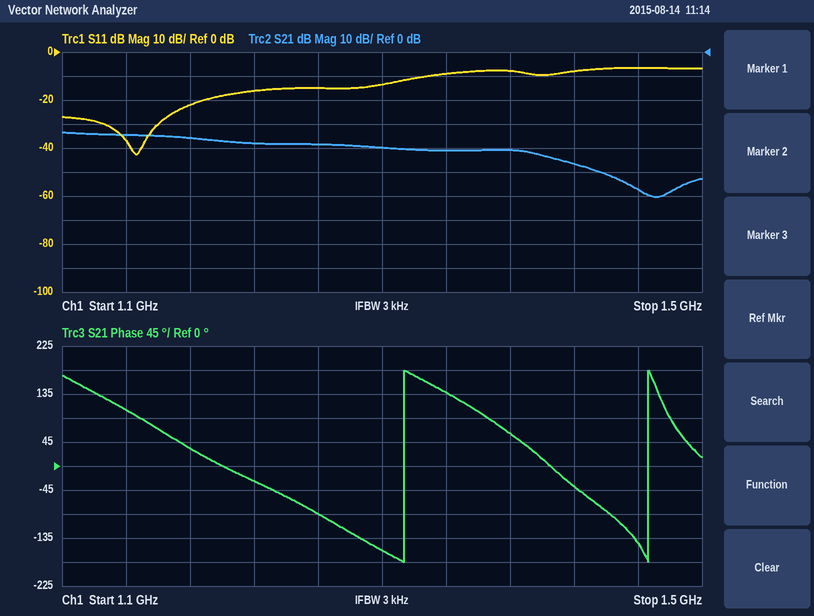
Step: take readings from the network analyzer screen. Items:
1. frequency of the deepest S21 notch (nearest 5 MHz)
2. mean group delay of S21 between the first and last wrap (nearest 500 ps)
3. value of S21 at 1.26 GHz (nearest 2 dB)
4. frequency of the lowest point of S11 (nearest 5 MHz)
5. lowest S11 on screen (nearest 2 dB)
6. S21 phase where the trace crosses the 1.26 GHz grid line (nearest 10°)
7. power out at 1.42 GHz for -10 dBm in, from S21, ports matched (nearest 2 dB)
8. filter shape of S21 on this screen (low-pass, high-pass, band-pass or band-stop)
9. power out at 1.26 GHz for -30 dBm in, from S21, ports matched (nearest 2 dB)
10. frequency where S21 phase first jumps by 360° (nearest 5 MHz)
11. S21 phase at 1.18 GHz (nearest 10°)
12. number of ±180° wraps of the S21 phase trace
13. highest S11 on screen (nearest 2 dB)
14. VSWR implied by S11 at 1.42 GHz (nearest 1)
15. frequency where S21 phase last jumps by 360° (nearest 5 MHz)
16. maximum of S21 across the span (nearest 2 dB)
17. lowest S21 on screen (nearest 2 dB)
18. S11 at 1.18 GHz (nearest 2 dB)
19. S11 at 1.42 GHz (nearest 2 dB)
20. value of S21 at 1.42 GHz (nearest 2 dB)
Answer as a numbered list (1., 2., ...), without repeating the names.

1. 1.470 GHz
2. 6.5 ns
3. -38 dB
4. 1.145 GHz
5. -42 dB
6. -90°
7. -56 dBm
8. low-pass
9. -68 dBm
10. 1.315 GHz
11. 30°
12. 2
13. -6 dB
14. 2
15. 1.465 GHz
16. -34 dB
17. -60 dB
18. -22 dB
19. -8 dB
20. -46 dB
